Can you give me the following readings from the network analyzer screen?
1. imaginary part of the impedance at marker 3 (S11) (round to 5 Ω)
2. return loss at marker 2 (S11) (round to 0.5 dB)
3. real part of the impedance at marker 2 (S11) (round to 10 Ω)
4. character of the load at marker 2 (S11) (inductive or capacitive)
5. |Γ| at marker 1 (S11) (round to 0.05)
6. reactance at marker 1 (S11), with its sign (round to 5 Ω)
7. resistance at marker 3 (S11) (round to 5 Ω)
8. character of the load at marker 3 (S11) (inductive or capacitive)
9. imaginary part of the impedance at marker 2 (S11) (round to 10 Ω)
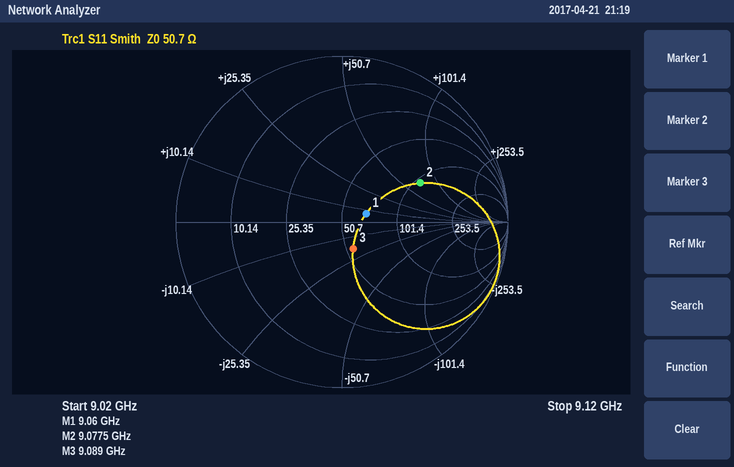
-20 Ω
5.5 dB
110 Ω
inductive
0.15
+5 Ω
55 Ω
capacitive
+70 Ω
